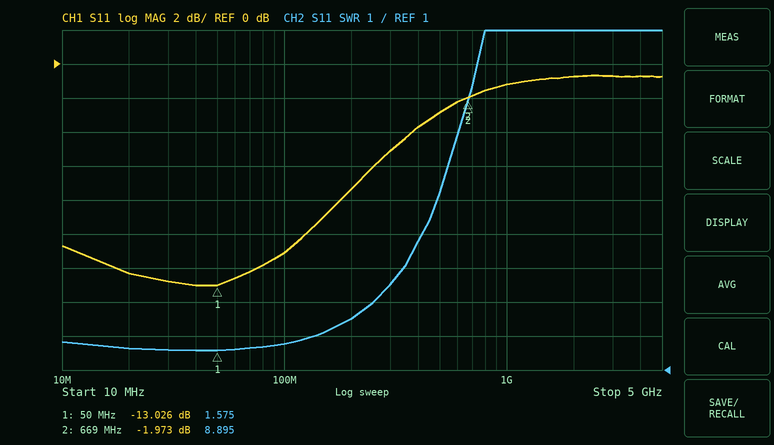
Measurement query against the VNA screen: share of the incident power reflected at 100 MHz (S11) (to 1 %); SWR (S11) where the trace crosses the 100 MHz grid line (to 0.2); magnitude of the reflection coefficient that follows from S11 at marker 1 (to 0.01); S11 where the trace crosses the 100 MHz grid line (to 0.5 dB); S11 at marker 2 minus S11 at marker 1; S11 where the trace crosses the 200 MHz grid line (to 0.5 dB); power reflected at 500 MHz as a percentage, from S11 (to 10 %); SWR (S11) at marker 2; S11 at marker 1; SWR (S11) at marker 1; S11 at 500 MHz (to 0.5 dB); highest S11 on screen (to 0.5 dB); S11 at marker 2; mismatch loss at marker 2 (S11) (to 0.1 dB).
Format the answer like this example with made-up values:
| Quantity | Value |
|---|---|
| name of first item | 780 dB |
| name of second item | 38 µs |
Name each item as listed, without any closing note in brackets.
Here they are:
| Quantity | Value |
|---|---|
| share of the incident power reflected at 100 MHz (S11) | 8 % |
| SWR (S11) where the trace crosses the 100 MHz grid line | 1.8 |
| magnitude of the reflection coefficient that follows from S11 at marker 1 | 0.22 |
| S11 where the trace crosses the 100 MHz grid line | -11.0 dB |
| S11 at marker 2 minus S11 at marker 1 | 11.053 dB |
| S11 where the trace crosses the 200 MHz grid line | -7.5 dB |
| power reflected at 500 MHz as a percentage, from S11 | 50 % |
| SWR (S11) at marker 2 | 8.895 |
| S11 at marker 1 | -13.026 dB |
| SWR (S11) at marker 1 | 1.575 |
| S11 at 500 MHz | -3.0 dB |
| highest S11 on screen | -0.5 dB |
| S11 at marker 2 | -1.973 dB |
| mismatch loss at marker 2 (S11) | 4.4 dB |
